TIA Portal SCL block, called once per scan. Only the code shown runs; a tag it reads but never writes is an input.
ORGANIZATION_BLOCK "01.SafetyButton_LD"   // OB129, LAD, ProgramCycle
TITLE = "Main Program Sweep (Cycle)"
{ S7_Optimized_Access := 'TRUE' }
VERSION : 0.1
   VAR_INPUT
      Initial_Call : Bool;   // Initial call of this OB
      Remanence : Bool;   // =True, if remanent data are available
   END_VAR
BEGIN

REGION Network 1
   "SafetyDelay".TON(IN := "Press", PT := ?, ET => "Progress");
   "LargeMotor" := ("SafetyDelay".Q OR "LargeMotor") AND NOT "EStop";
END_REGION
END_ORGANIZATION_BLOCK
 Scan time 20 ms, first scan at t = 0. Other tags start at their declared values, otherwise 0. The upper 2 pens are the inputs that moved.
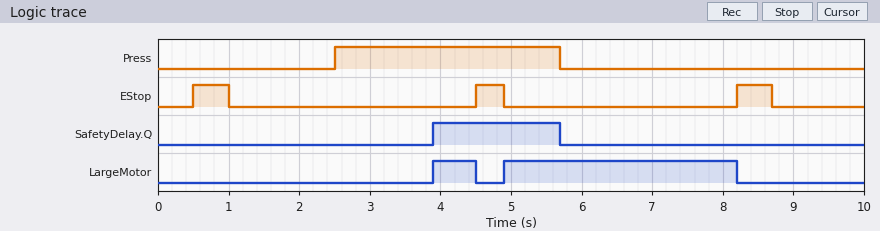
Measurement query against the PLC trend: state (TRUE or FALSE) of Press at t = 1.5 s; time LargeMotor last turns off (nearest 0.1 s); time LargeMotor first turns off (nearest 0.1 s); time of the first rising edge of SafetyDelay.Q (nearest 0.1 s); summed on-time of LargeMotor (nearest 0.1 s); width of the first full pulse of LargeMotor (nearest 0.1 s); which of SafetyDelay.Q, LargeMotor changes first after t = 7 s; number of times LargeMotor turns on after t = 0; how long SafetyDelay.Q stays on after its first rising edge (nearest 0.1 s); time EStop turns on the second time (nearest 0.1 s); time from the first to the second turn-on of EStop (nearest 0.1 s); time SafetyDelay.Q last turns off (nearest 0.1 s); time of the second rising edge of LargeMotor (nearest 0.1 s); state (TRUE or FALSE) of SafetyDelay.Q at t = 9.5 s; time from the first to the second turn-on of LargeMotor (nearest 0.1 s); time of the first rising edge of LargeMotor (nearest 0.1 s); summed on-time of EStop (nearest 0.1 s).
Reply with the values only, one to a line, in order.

FALSE
8.2 s
4.5 s
3.9 s
3.9 s
0.6 s
LargeMotor
2
1.8 s
4.5 s
4.0 s
5.7 s
4.9 s
FALSE
1.0 s
3.9 s
1.4 s
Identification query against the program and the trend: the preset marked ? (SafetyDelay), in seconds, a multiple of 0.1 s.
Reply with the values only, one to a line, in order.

1.4 s
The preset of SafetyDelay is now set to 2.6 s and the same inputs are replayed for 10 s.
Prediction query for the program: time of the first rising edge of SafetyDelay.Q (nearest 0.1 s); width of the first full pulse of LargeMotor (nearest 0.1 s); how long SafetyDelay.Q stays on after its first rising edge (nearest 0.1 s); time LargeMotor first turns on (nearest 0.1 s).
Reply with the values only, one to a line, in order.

5.1 s
3.1 s
0.6 s
5.1 s
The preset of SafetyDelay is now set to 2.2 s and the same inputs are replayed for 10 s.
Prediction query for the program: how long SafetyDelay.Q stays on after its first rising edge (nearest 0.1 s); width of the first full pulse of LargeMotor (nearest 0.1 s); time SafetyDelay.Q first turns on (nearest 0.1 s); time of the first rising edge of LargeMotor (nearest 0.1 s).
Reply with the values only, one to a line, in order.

1.0 s
3.3 s
4.7 s
4.9 s
